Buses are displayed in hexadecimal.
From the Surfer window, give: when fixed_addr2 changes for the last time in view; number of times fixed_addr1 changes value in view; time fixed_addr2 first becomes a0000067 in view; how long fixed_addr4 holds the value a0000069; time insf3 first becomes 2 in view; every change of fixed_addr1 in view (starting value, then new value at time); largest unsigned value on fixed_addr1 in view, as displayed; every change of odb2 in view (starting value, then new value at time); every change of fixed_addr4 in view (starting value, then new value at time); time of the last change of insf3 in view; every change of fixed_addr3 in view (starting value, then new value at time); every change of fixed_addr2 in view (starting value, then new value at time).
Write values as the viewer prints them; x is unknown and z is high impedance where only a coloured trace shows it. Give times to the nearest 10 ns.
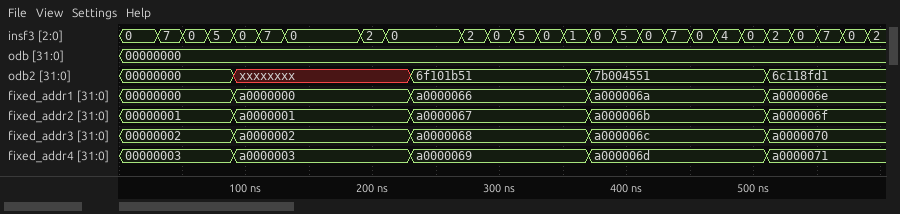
510 ns
4
230 ns
140 ns
190 ns
00000000, a0000000 at 90 ns, a0000066 at 230 ns, a000006a at 370 ns, a000006e at 510 ns
a000006e
00000000, xxxxxxxx at 90 ns, 6f101b51 at 230 ns, 7b004551 at 370 ns, 6c118fd1 at 510 ns
00000003, a0000003 at 90 ns, a0000069 at 230 ns, a000006d at 370 ns, a0000071 at 510 ns
590 ns
00000002, a0000002 at 90 ns, a0000068 at 230 ns, a000006c at 370 ns, a0000070 at 510 ns
00000001, a0000001 at 90 ns, a0000067 at 230 ns, a000006b at 370 ns, a000006f at 510 ns
